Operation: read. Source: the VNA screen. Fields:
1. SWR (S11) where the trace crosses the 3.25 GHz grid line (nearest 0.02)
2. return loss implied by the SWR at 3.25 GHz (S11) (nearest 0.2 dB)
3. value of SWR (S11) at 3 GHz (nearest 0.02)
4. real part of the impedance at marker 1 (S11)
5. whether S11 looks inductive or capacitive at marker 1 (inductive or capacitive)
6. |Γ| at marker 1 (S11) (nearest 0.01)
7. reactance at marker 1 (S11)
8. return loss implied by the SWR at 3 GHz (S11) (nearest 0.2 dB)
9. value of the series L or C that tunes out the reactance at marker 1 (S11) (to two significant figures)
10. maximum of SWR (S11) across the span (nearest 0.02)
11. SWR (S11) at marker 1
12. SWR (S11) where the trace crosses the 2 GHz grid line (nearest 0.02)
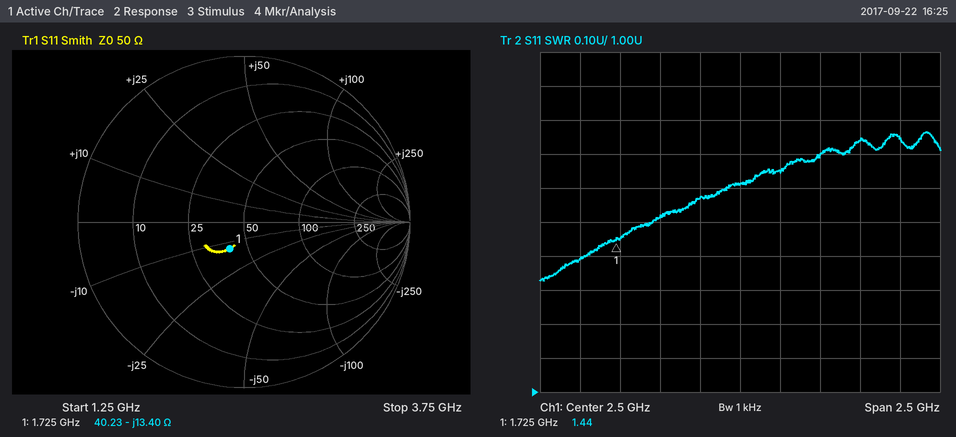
1.74
11.4 dB
1.70
40.23 Ω
capacitive
0.18
-13.40 Ω
11.8 dB
1.2 nH
1.76
1.44
1.52
